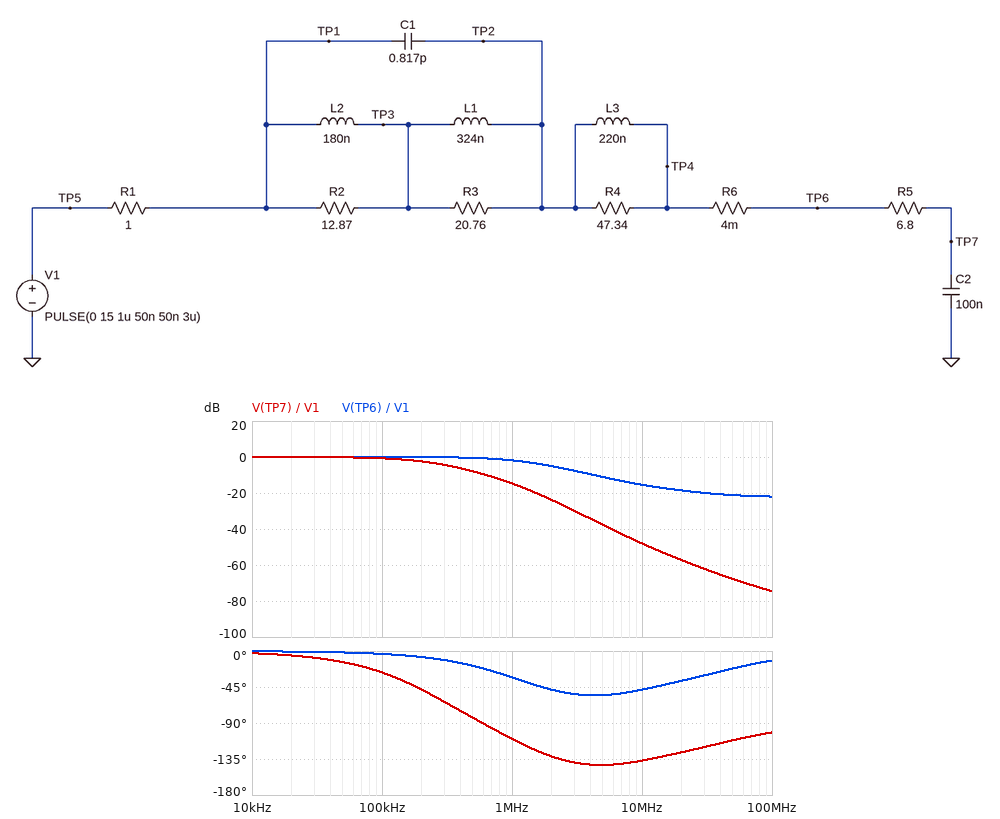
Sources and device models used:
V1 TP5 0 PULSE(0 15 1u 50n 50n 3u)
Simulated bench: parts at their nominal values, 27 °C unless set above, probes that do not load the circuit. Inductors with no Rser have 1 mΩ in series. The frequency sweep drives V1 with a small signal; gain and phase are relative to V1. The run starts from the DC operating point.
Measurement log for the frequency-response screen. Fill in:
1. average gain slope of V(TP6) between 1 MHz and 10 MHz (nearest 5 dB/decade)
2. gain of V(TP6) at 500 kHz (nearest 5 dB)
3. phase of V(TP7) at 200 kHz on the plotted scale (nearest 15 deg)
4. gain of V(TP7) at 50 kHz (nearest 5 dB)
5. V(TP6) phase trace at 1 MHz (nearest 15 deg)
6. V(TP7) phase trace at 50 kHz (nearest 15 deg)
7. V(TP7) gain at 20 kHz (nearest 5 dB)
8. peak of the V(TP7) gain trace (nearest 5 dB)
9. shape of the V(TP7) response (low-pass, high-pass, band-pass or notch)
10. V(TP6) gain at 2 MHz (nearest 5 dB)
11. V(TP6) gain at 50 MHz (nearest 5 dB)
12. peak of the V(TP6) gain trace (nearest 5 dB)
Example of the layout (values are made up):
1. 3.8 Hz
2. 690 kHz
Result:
1. -15 dB/decade
2. 0 dB
3. -45 deg
4. 0 dB
5. -30 deg
6. -15 deg
7. 0 dB
8. 0 dB
9. low-pass
10. -5 dB
11. -20 dB
12. 0 dB
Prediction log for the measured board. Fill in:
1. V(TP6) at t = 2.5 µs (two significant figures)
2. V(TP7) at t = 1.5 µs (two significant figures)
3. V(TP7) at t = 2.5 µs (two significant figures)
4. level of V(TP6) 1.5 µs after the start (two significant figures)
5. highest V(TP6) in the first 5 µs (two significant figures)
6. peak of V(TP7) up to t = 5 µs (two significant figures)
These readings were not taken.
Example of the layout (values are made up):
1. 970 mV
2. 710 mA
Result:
1. 15 V
2. 6.2 V
3. 13 V
4. 15 V
5. 15 V
6. 15 V
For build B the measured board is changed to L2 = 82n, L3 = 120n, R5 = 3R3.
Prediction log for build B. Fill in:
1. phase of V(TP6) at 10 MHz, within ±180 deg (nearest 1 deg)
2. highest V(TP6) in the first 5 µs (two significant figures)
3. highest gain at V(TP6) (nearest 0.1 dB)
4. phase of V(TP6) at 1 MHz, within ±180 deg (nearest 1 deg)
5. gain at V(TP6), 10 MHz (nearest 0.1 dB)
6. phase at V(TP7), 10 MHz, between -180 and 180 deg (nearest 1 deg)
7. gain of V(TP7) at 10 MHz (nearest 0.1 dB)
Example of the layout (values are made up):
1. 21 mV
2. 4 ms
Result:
1. -54 deg
2. 16 V
3. 0.2 dB
4. -46 deg
5. -18.6 dB
6. -142 deg
7. -44.9 dB
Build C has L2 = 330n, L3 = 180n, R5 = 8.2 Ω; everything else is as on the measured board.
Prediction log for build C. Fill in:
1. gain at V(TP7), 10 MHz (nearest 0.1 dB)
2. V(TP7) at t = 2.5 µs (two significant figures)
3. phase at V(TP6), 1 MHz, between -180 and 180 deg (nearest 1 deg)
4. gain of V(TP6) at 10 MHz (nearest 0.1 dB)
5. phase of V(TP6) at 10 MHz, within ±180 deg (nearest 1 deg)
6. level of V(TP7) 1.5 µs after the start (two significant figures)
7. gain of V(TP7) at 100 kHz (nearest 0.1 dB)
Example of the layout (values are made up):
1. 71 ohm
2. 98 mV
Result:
1. -48.2 dB
2. 12 V
3. -31 deg
4. -14.0 dB
5. -42 deg
6. 5.4 V
7. -1.0 dB
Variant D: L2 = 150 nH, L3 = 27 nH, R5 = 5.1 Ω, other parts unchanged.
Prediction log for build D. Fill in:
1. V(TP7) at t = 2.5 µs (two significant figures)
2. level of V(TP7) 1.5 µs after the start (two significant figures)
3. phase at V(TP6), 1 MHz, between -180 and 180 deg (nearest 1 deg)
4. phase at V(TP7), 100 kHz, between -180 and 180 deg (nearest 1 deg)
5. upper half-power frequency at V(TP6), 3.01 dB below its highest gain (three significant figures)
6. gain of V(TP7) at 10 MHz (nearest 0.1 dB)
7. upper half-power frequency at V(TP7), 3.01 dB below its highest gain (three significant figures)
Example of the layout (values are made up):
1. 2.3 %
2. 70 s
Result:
1. 14 V
2. 7.6 V
3. -31 deg
4. -21 deg
5. 1.41 MHz
6. -44.8 dB
7. 298 kHz
